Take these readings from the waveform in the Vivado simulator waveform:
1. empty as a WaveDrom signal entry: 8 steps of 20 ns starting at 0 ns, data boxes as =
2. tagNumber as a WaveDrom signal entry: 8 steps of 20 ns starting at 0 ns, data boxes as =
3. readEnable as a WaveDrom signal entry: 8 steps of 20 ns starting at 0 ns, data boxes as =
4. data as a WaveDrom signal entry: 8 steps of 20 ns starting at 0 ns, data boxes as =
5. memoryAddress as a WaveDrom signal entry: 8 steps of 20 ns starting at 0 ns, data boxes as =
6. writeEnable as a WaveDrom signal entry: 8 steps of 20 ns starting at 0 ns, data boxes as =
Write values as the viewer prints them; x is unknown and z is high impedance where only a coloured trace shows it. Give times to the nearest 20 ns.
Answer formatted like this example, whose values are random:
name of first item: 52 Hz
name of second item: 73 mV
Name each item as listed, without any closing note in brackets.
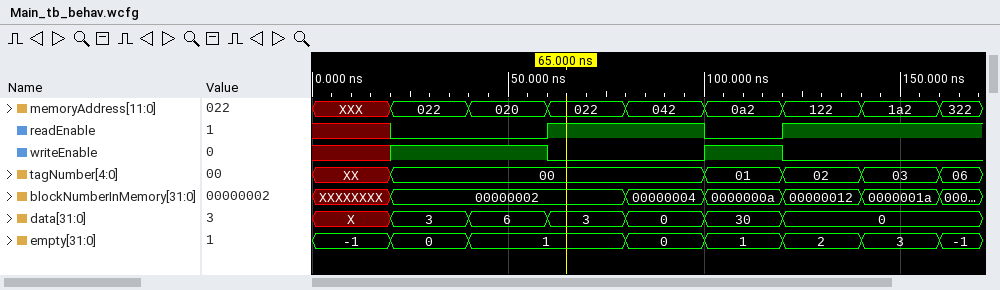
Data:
empty as a WaveDrom signal entry: 8 steps of 20 ns starting at 0 ns, data boxes as =: {name: 'empty', wave: '===.====', data: '-1 0 1 0 1 2 3'}
tagNumber as a WaveDrom signal entry: 8 steps of 20 ns starting at 0 ns, data boxes as =: {name: 'tagNumber', wave: 'x=...===', data: '00 01 02 03'}
readEnable as a WaveDrom signal entry: 8 steps of 20 ns starting at 0 ns, data boxes as =: {name: 'readEnable', wave: 'x0.1.01.'}
data as a WaveDrom signal entry: 8 steps of 20 ns starting at 0 ns, data boxes as =: {name: 'data', wave: 'x======.', data: '3 6 3 0 30 0'}
memoryAddress as a WaveDrom signal entry: 8 steps of 20 ns starting at 0 ns, data boxes as =: {name: 'memoryAddress', wave: 'x=======', data: '022 020 022 042 0a2 122 1a2'}
writeEnable as a WaveDrom signal entry: 8 steps of 20 ns starting at 0 ns, data boxes as =: {name: 'writeEnable', wave: 'x1.0.10.'}
